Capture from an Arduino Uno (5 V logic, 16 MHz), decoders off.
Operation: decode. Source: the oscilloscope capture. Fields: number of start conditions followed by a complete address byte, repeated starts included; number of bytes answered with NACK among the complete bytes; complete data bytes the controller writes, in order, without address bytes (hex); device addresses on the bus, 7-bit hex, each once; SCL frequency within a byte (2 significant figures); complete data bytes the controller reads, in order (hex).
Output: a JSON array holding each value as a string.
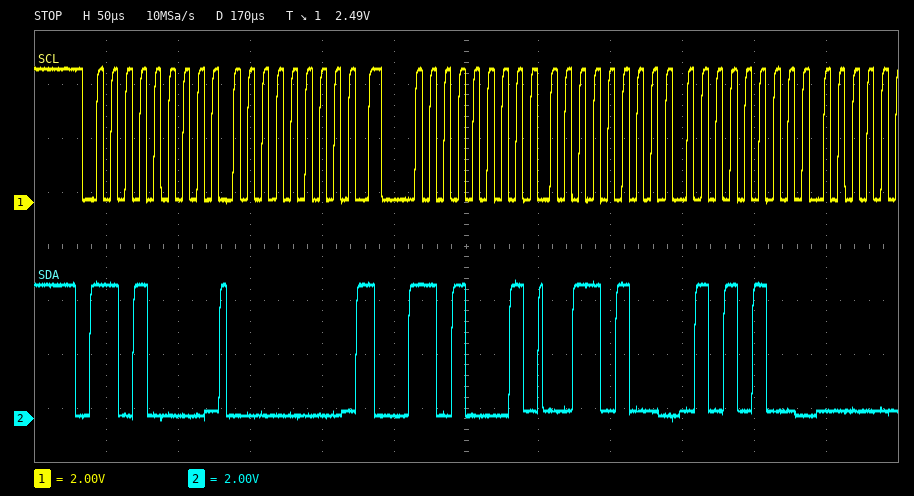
["2", "0", "00", "0x68", "100 kHz", "34 54"]
